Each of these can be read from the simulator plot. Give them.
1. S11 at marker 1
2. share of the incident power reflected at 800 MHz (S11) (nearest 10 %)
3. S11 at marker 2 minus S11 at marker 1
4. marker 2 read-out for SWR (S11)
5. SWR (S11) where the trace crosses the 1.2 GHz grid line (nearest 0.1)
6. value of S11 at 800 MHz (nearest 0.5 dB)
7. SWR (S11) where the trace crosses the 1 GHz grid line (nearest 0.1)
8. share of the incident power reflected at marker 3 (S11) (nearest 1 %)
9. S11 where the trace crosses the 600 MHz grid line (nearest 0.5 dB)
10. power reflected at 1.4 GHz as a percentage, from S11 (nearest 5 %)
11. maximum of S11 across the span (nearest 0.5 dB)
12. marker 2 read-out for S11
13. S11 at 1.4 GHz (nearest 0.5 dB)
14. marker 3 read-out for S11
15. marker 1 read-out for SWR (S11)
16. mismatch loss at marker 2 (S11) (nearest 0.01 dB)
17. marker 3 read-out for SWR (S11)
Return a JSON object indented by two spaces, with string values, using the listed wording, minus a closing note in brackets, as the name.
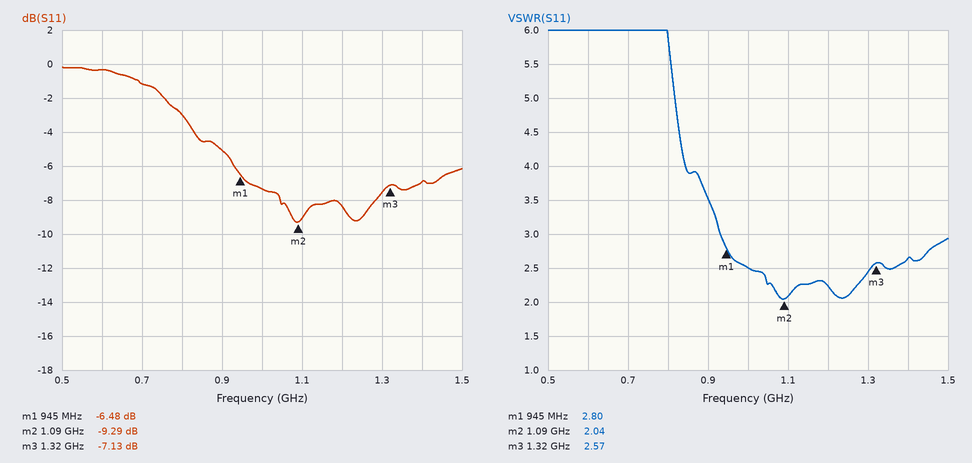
{
  "S11 at marker 1": "-6.48 dB",
  "share of the incident power reflected at 800 MHz (S11)": "50 %",
  "S11 at marker 2 minus S11 at marker 1": "-2.81 dB",
  "marker 2 read-out for SWR": "2.04",
  "SWR (S11) where the trace crosses the 1.2 GHz grid line": "2.2",
  "value of S11 at 800 MHz": "-3.0 dB",
  "SWR (S11) where the trace crosses the 1 GHz grid line": "2.5",
  "share of the incident power reflected at marker 3 (S11)": "19 %",
  "S11 where the trace crosses the 600 MHz grid line": "-0.5 dB",
  "power reflected at 1.4 GHz as a percentage, from S11": "20 %",
  "maximum of S11 across the span": "0.0 dB",
  "marker 2 read-out for S11": "-9.29 dB",
  "S11 at 1.4 GHz": "-7.0 dB",
  "marker 3 read-out for S11": "-7.13 dB",
  "marker 1 read-out for SWR": "2.80",
  "mismatch loss at marker 2 (S11)": "0.54 dB",
  "marker 3 read-out for SWR": "2.57"
}
